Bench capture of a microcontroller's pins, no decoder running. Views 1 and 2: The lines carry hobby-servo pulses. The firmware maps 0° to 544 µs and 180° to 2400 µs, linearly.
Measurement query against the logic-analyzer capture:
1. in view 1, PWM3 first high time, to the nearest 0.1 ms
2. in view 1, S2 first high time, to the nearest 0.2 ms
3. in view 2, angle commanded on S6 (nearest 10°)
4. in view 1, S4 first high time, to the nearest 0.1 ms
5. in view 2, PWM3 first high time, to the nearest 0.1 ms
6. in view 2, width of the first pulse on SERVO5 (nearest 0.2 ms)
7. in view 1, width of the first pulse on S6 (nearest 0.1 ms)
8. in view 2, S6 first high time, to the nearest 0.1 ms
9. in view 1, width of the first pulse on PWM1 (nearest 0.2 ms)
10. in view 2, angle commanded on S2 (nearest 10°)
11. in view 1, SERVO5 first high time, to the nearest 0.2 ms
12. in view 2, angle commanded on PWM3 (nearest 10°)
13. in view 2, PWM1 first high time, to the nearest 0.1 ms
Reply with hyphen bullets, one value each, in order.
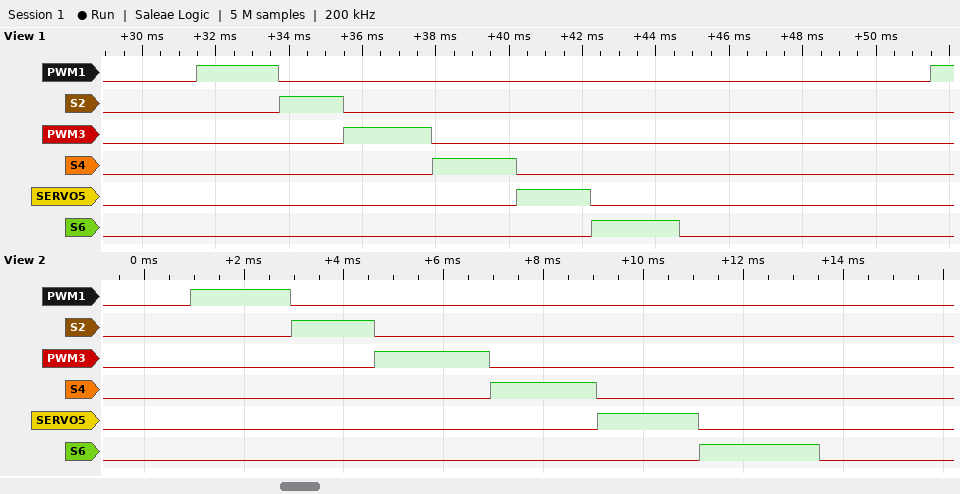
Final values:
- 2.4 ms
- 1.8 ms
- 180°
- 2.3 ms
- 2.3 ms
- 2.0 ms
- 2.4 ms
- 2.4 ms
- 2.2 ms
- 110°
- 2.0 ms
- 170°
- 2.0 ms
